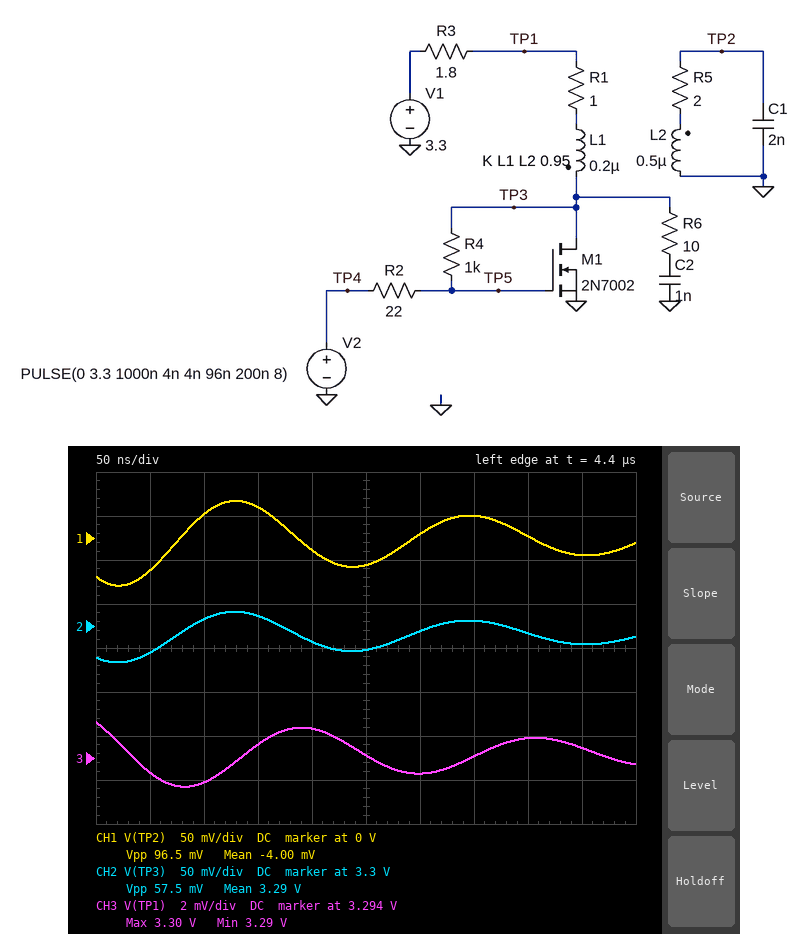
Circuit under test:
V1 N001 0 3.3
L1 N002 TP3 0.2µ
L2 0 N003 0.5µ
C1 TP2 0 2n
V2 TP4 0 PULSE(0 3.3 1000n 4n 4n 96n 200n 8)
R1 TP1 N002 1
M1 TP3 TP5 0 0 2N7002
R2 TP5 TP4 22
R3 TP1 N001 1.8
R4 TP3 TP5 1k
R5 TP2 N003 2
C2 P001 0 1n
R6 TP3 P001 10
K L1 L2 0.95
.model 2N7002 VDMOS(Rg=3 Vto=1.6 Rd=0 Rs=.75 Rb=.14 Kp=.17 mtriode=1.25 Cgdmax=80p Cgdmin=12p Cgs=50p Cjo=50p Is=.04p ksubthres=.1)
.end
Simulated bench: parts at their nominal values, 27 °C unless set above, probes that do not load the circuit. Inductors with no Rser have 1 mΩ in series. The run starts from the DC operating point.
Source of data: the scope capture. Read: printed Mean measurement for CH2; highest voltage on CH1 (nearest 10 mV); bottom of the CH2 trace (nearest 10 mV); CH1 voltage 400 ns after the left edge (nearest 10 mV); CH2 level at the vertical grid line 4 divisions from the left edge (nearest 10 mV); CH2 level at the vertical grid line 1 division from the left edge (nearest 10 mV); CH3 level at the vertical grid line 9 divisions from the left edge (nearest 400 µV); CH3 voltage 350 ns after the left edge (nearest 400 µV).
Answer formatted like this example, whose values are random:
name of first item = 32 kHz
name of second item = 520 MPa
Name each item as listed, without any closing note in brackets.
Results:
printed Mean measurement for CH2 = 3.29 V
highest voltage on CH1 = 40 mV
bottom of the CH2 trace = 3.26 V
CH1 voltage 400 ns after the left edge = 0 V
CH2 level at the vertical grid line 4 divisions from the left edge = 3.28 V
CH2 level at the vertical grid line 1 division from the left edge = 3.27 V
CH3 level at the vertical grid line 9 divisions from the left edge = 3.2944 V
CH3 voltage 350 ns after the left edge = 3.2940 V
